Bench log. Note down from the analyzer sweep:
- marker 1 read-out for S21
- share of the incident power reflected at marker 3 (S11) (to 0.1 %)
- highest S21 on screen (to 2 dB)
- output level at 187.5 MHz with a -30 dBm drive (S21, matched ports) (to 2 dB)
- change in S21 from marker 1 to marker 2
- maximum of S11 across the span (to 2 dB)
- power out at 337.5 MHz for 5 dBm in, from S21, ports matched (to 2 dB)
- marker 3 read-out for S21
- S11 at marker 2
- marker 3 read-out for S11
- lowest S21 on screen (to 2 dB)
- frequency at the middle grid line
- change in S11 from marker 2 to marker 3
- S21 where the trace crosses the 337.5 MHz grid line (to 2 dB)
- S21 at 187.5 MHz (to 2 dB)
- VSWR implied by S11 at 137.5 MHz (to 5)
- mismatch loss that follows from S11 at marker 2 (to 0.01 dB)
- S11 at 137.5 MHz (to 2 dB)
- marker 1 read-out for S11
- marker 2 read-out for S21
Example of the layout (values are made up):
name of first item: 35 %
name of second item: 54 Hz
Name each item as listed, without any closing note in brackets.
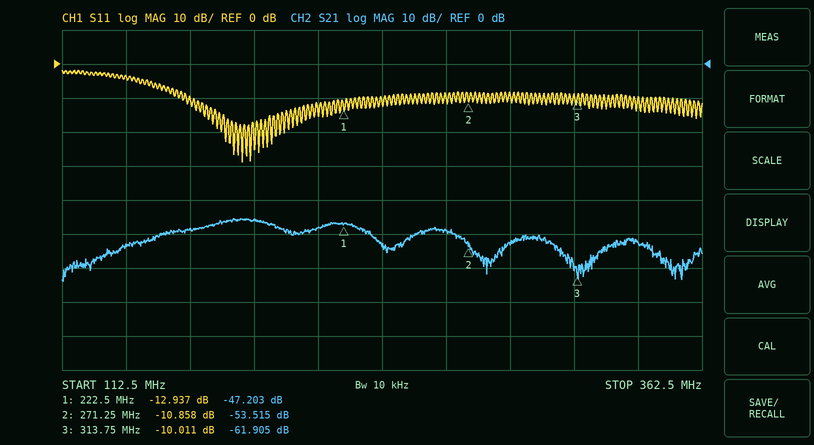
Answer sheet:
marker 1 read-out for S21: -47.203 dB
share of the incident power reflected at marker 3 (S11): 10.0 %
highest S21 on screen: -46 dB
output level at 187.5 MHz with a -30 dBm drive (S21, matched ports): -76 dBm
change in S21 from marker 1 to marker 2: -6.312 dB
maximum of S11 across the span: -2 dB
power out at 337.5 MHz for 5 dBm in, from S21, ports matched: -48 dBm
marker 3 read-out for S21: -61.905 dB
S11 at marker 2: -10.858 dB
marker 3 read-out for S11: -10.011 dB
lowest S21 on screen: -64 dB
frequency at the middle grid line: 237.5 MHz
change in S11 from marker 2 to marker 3: 0.847 dB
S21 where the trace crosses the 337.5 MHz grid line: -52 dB
S21 at 187.5 MHz: -46 dB
VSWR implied by S11 at 137.5 MHz: 5
mismatch loss that follows from S11 at marker 2: 0.37 dB
S11 at 137.5 MHz: -4 dB
marker 1 read-out for S11: -12.937 dB
marker 2 read-out for S21: -53.515 dB
